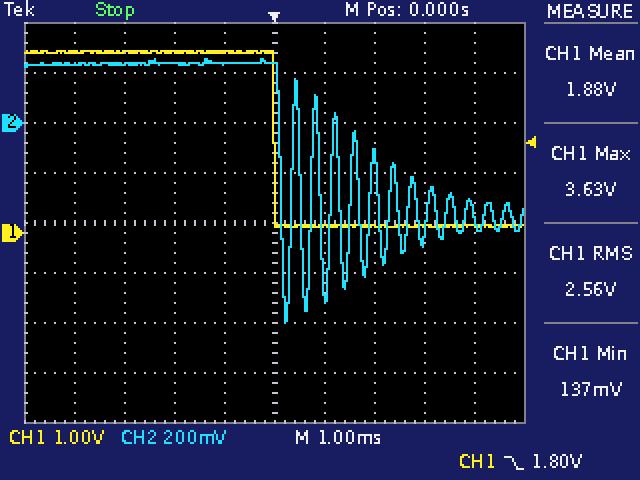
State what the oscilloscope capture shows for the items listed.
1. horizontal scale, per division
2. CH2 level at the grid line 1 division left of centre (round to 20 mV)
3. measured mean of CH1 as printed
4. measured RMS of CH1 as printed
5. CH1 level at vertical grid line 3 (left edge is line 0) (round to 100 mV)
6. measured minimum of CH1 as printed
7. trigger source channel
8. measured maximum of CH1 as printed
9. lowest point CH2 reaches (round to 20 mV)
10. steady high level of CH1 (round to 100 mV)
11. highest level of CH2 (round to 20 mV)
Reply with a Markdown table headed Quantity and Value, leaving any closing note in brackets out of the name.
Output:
| Quantity | Value |
|---|---|
| horizontal scale, per division | 1 ms |
| CH2 level at the grid line 1 division left of centre | 240 mV |
| measured mean of CH1 as printed | 1.88 V |
| measured RMS of CH1 as printed | 2.56 V |
| CH1 level at vertical grid line 3 (left edge is line 0) | 3.6 V |
| measured minimum of CH1 as printed | 137 mV |
| trigger source channel | CH1 |
| measured maximum of CH1 as printed | 3.63 V |
| lowest point CH2 reaches | -800 mV |
| steady high level of CH1 | 3.6 V |
| highest level of CH2 | 260 mV |
